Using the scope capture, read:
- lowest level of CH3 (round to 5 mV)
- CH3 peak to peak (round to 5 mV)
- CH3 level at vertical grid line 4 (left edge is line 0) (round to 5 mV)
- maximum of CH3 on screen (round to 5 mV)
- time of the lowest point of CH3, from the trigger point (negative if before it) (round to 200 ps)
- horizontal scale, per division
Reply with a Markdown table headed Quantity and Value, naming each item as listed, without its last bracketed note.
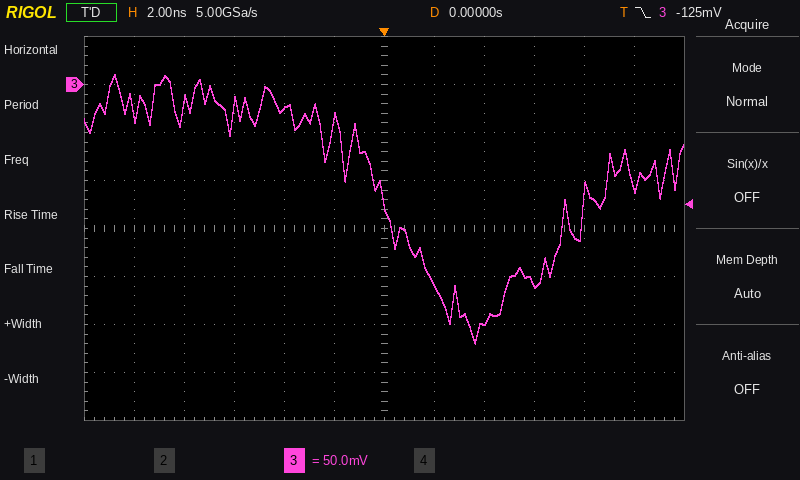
| Quantity | Value |
|---|---|
| lowest level of CH3 | -270 mV |
| CH3 peak to peak | 280 mV |
| CH3 level at vertical grid line 4 (left edge is line 0) | -25 mV |
| maximum of CH3 on screen | 10 mV |
| time of the lowest point of CH3, from the trigger point (negative if before it) | +3.6 ns |
| horizontal scale, per division | 2 ns |
